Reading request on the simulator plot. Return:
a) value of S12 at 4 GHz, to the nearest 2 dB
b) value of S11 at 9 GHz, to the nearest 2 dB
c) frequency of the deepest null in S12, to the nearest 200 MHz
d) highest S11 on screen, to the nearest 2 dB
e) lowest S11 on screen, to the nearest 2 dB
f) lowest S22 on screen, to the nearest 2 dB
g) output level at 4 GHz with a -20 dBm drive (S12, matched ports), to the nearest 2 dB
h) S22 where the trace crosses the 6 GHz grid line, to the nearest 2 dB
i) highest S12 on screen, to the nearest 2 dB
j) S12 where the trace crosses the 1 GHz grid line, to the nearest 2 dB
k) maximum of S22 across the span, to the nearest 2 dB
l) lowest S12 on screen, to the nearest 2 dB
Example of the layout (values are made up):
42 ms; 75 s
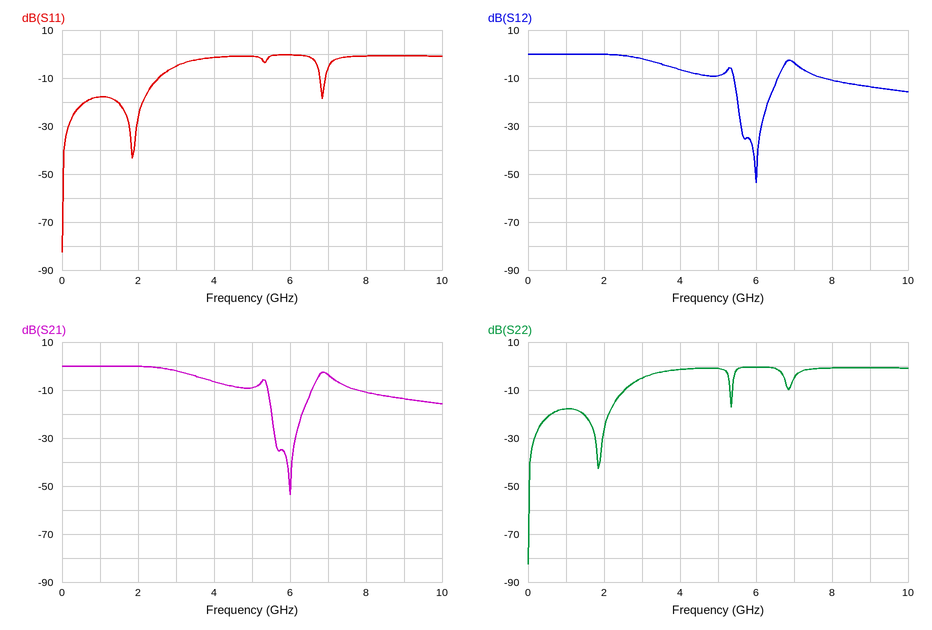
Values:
-6 dB; 0 dB; 6.0 GHz; 0 dB; -82 dB; -82 dB; -26 dBm; 0 dB; 0 dB; 0 dB; 0 dB; -54 dB
